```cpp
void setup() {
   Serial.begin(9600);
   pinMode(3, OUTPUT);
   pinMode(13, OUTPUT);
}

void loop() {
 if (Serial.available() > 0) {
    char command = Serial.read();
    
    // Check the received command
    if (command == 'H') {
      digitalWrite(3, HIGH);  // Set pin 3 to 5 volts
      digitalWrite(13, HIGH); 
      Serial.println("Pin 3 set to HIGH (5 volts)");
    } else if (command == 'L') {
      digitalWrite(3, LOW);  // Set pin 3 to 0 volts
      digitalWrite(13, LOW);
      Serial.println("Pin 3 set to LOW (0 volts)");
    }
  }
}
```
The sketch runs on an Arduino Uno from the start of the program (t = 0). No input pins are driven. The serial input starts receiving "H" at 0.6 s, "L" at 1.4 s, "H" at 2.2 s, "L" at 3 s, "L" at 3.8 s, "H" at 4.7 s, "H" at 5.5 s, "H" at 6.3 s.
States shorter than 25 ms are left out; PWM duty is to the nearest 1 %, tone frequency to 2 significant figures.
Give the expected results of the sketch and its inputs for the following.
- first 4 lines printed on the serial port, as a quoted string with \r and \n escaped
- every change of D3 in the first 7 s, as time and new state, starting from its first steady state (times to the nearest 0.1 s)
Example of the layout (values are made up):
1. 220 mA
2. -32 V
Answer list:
1. "Pin 3 set to HIGH (5 volts)\r\nPin 3 set to LOW (0 volts)\r\nPin 3 set to HIGH (5 volts)\r\nPin 3 set to LOW (0 volts)\r\n"
2. 0 s low; 0.6 s high; 1.4 s low; 2.2 s high; 3 s low; 4.7 s high
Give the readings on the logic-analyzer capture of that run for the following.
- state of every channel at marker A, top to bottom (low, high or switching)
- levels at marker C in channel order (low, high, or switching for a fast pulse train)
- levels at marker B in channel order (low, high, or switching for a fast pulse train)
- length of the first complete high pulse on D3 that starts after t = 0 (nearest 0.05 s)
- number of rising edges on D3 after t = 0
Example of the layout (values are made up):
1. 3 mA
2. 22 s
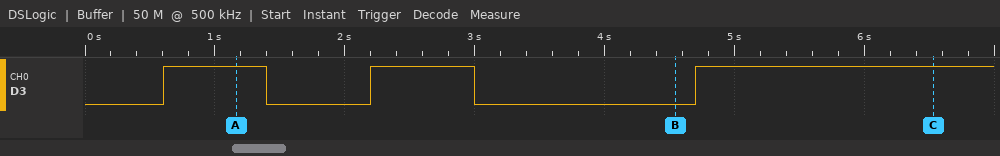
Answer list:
1. D3 high
2. D3 high
3. D3 low
4. 0.80 s
5. 3
